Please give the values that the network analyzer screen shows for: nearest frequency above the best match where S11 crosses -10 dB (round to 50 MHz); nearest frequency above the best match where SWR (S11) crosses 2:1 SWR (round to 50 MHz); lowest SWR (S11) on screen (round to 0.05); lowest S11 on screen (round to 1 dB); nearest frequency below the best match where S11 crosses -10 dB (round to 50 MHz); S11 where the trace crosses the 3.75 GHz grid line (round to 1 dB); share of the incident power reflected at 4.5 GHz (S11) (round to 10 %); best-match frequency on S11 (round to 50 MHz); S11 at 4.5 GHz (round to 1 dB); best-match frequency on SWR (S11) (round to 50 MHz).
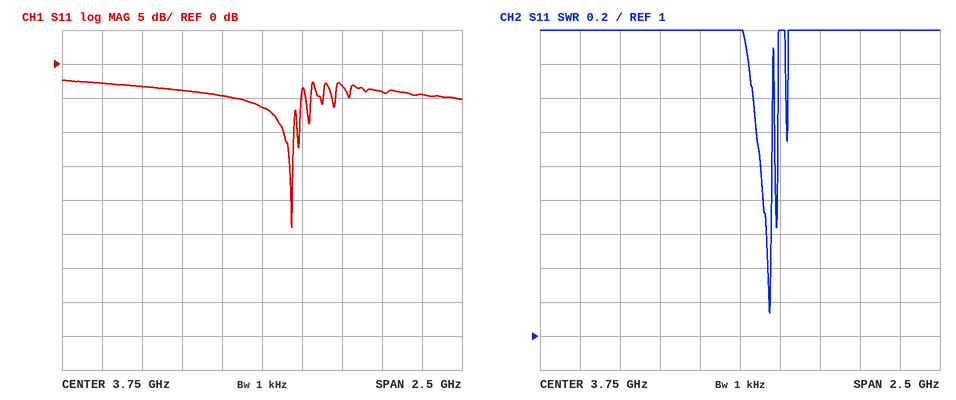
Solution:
3.95 GHz
3.95 GHz
1.15
-24 dB
3.90 GHz
-6 dB
40 %
3.95 GHz
-4 dB
3.95 GHz
